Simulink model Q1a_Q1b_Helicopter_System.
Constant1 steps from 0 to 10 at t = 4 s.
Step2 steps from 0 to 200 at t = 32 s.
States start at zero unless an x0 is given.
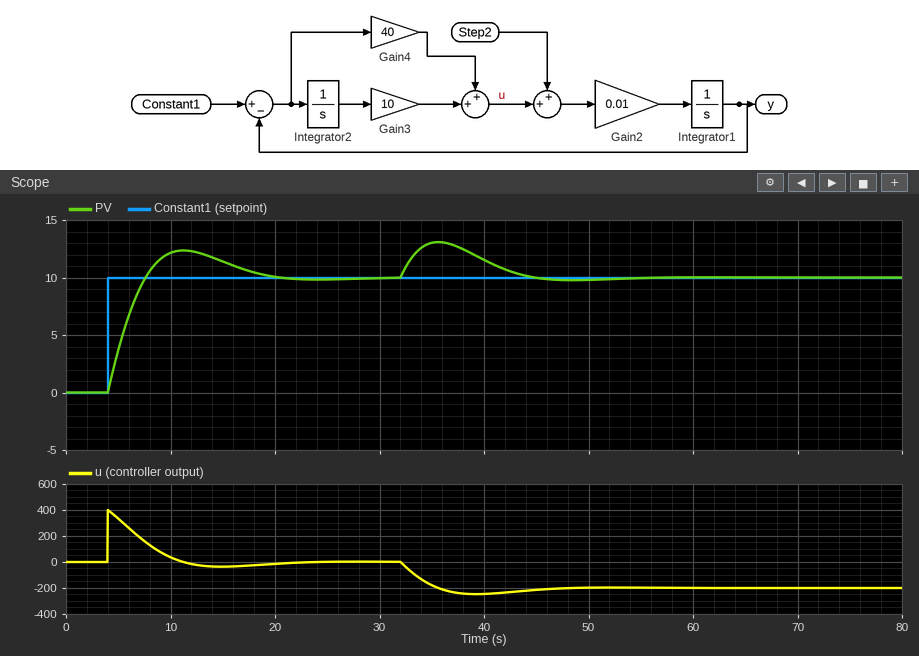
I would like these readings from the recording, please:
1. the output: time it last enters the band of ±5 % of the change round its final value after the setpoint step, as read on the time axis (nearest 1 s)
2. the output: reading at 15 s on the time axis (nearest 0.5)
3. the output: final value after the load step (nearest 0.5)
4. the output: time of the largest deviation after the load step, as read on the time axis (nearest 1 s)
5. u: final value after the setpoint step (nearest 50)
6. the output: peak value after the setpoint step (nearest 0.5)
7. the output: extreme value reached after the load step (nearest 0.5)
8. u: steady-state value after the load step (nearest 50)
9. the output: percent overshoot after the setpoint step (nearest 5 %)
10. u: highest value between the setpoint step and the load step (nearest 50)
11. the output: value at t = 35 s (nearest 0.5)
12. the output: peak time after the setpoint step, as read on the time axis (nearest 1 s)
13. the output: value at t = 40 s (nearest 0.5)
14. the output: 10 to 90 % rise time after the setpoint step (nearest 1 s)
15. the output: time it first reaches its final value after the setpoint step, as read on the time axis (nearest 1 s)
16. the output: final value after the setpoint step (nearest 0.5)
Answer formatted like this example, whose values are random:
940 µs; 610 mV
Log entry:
18 s; 11.5; 10.0; 36 s; 0; 12.5; 13.0; -200; 25 %; 400; 13.0; 11 s; 11.5; 3 s; 8 s; 10.0
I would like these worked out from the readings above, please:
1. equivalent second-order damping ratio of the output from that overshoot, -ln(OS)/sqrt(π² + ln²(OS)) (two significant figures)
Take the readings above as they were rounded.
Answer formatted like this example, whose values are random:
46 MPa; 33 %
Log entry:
0.40
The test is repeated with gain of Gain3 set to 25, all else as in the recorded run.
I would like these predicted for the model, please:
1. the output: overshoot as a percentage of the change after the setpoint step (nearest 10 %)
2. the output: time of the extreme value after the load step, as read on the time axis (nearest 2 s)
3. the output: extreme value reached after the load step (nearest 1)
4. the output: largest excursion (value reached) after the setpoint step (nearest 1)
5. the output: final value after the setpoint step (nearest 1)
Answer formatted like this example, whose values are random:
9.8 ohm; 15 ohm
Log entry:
40 %; 34 s; 12; 14; 10
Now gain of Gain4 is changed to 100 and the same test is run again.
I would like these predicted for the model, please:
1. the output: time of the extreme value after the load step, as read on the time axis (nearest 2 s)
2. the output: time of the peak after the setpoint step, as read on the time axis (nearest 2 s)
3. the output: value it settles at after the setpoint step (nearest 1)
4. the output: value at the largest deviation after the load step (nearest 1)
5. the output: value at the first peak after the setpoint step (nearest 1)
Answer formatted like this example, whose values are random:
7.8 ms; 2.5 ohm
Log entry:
34 s; 10 s; 10; 12; 11
